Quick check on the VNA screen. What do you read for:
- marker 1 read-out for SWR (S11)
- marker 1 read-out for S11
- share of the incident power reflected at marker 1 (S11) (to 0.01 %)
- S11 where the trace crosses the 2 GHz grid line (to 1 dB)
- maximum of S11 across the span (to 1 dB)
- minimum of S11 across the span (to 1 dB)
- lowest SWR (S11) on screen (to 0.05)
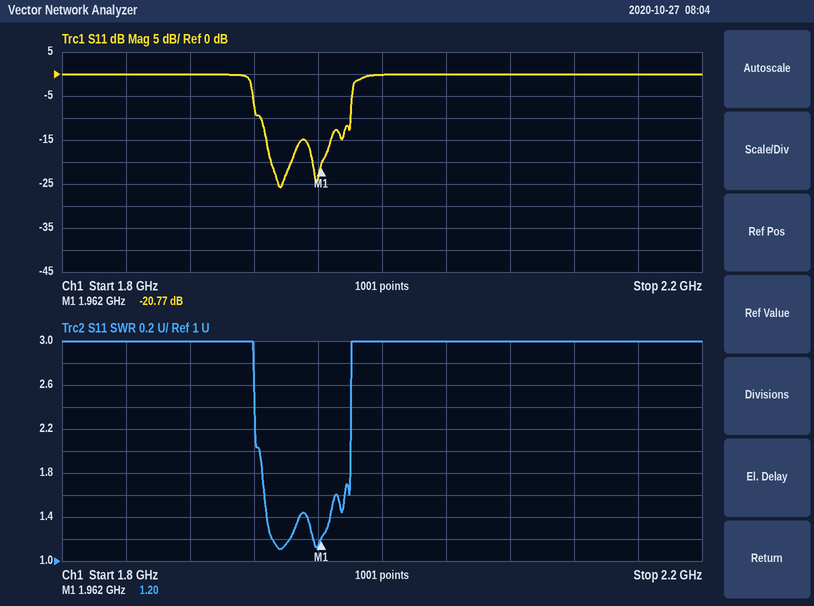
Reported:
1.20
-20.77 dB
0.84 %
0 dB
0 dB
-26 dB
1.10
